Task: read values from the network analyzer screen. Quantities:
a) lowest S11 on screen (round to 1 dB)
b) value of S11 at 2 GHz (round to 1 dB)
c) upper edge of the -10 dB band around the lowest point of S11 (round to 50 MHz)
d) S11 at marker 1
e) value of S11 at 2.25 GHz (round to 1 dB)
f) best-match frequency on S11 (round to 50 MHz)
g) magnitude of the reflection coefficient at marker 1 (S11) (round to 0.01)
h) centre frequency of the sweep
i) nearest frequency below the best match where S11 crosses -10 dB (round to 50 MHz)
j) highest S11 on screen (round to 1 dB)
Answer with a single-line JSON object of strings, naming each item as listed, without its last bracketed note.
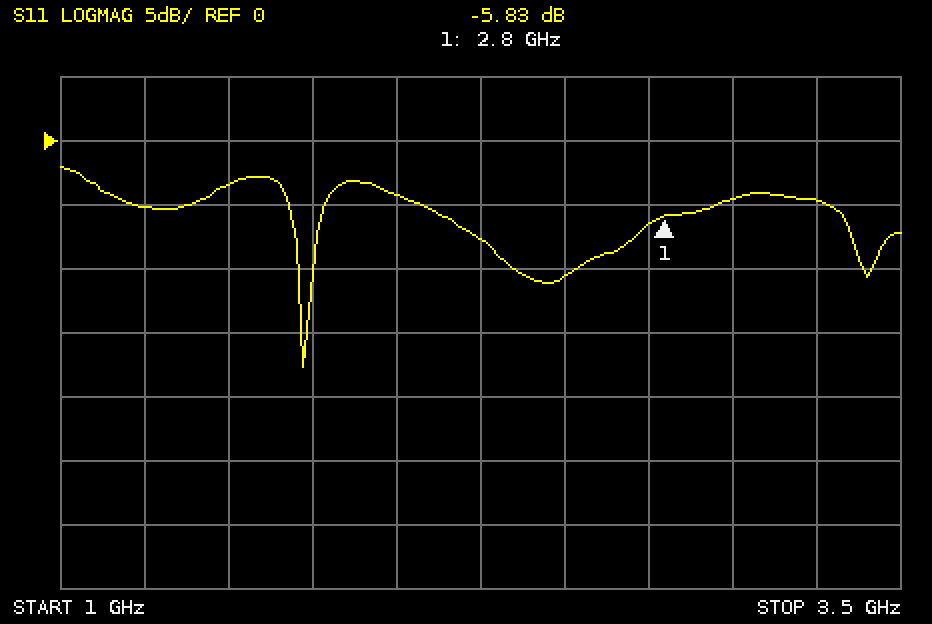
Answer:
{"lowest S11 on screen": "-18 dB", "value of S11 at 2 GHz": "-4 dB", "upper edge of the -10 dB band around the lowest point of S11": "1.75 GHz", "S11 at marker 1": "-5.83 dB", "value of S11 at 2.25 GHz": "-8 dB", "best-match frequency on S11": "1.70 GHz", "magnitude of the reflection coefficient at marker 1 (S11)": "0.51", "centre frequency of the sweep": "2.25 GHz", "nearest frequency below the best match where S11 crosses -10 dB": "1.70 GHz", "highest S11 on screen": "-2 dB"}
